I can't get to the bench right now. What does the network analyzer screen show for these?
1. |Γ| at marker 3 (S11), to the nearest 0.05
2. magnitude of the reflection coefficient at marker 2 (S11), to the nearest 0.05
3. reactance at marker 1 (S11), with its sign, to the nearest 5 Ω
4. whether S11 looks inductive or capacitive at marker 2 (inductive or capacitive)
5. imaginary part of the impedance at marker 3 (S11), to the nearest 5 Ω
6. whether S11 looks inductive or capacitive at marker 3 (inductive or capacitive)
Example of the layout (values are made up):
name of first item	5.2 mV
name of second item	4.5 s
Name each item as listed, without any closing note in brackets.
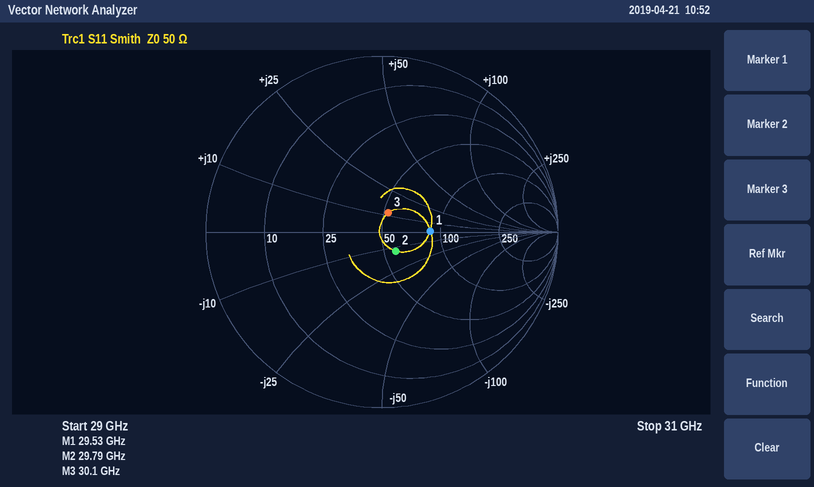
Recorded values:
|Γ| at marker 3 (S11), to the nearest 0.05	0.10
magnitude of the reflection coefficient at marker 2 (S11), to the nearest 0.05	0.15
reactance at marker 1 (S11), with its sign, to the nearest 5 Ω	0 Ω
whether S11 looks inductive or capacitive at marker 2	capacitive
imaginary part of the impedance at marker 3 (S11), to the nearest 5 Ω	+10 Ω
whether S11 looks inductive or capacitive at marker 3	inductive
